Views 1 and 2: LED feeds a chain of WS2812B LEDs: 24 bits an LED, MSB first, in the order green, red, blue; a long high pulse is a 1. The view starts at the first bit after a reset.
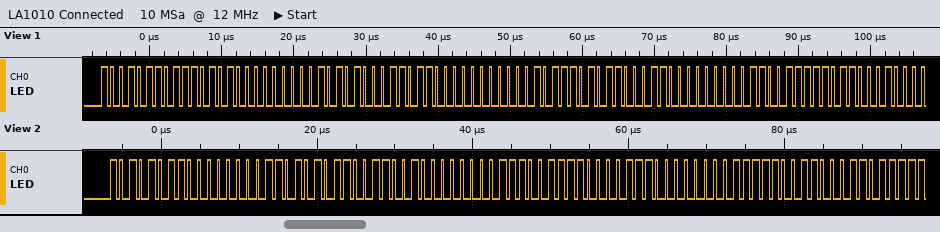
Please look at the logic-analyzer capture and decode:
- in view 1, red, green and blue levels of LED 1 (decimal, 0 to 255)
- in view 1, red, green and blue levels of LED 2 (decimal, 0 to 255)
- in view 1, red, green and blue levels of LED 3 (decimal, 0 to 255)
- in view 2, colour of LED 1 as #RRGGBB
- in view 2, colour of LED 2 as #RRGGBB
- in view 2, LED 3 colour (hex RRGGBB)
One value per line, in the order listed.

234, 150, 0
216, 168, 0
198, 186, 0
#00ABD5
#0099E7
#0087F9
